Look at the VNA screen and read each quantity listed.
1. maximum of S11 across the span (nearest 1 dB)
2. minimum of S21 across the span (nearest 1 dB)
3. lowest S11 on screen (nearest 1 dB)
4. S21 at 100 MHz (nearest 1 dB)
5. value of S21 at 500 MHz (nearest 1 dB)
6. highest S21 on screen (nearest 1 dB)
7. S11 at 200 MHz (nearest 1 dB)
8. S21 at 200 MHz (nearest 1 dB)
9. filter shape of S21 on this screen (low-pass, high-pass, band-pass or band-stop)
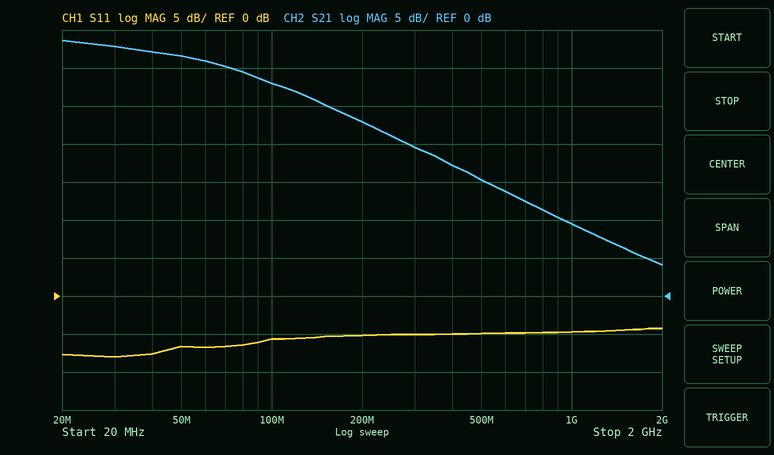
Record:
-4 dB
4 dB
-8 dB
28 dB
15 dB
34 dB
-5 dB
23 dB
low-pass
